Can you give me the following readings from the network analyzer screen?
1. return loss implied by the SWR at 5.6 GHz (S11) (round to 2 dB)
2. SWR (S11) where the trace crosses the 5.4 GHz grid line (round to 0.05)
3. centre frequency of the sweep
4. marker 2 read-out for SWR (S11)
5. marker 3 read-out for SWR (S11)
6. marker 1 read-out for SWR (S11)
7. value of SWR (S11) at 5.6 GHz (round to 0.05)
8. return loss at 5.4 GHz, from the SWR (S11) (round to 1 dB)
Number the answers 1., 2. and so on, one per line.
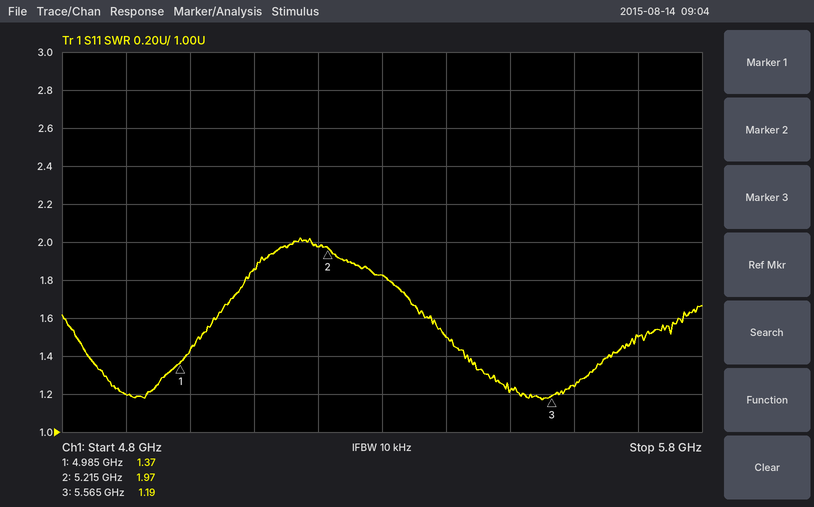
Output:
1. 20 dB
2. 1.50
3. 5.3 GHz
4. 1.97
5. 1.19
6. 1.37
7. 1.25
8. 14 dB
